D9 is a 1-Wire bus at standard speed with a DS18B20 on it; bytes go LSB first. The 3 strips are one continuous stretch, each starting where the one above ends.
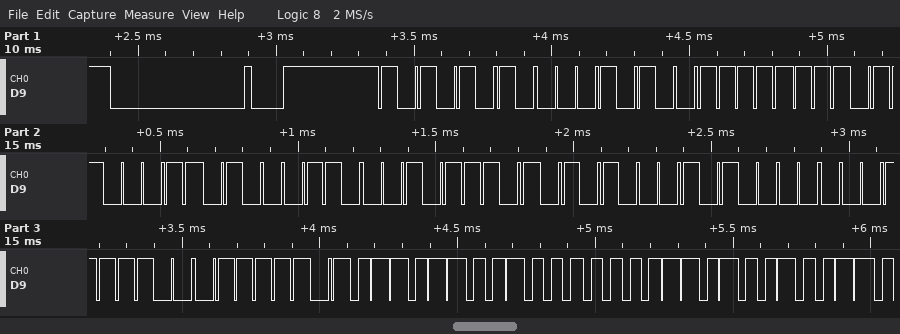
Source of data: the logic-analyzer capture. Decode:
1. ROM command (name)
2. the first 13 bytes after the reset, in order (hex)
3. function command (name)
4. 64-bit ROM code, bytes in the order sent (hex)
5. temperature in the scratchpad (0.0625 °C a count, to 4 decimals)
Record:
Match ROM
55 28 FF C6 62 74 15 05 3C BE 36 01 4B
Read Scratchpad
28 FF C6 62 74 15 05 3C
19.3750 °C
